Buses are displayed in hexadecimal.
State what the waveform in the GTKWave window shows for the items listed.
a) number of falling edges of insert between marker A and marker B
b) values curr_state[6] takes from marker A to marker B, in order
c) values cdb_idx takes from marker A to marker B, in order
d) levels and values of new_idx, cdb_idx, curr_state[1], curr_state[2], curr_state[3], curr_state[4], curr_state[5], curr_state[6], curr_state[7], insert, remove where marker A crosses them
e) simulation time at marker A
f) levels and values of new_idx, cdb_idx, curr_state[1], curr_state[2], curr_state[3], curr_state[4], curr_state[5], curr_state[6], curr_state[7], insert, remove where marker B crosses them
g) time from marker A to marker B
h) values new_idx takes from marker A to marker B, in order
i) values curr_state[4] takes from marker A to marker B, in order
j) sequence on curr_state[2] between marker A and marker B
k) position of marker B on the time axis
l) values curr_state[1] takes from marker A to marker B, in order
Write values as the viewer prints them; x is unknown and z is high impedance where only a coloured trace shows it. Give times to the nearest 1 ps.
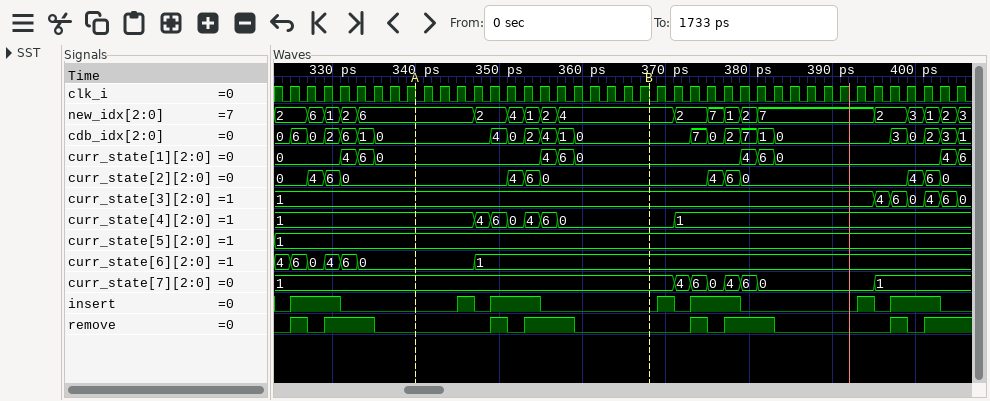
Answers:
2
0, 1
0, 4, 0, 2, 4, 1, 0
new_idx=6, cdb_idx=0, curr_state[1]=0, curr_state[2]=0, curr_state[3]=1, curr_state[4]=1, curr_state[5]=1, curr_state[6]=0, curr_state[7]=1, insert=0, remove=0
340 ps
new_idx=4, cdb_idx=0, curr_state[1]=0, curr_state[2]=0, curr_state[3]=1, curr_state[4]=0, curr_state[5]=1, curr_state[6]=1, curr_state[7]=1, insert=0, remove=0
28 ps
6, 2, 4, 1, 2, 4
1, 4, 6, 0, 4, 6, 0
0, 4, 6, 0
368 ps
0, 4, 6, 0
